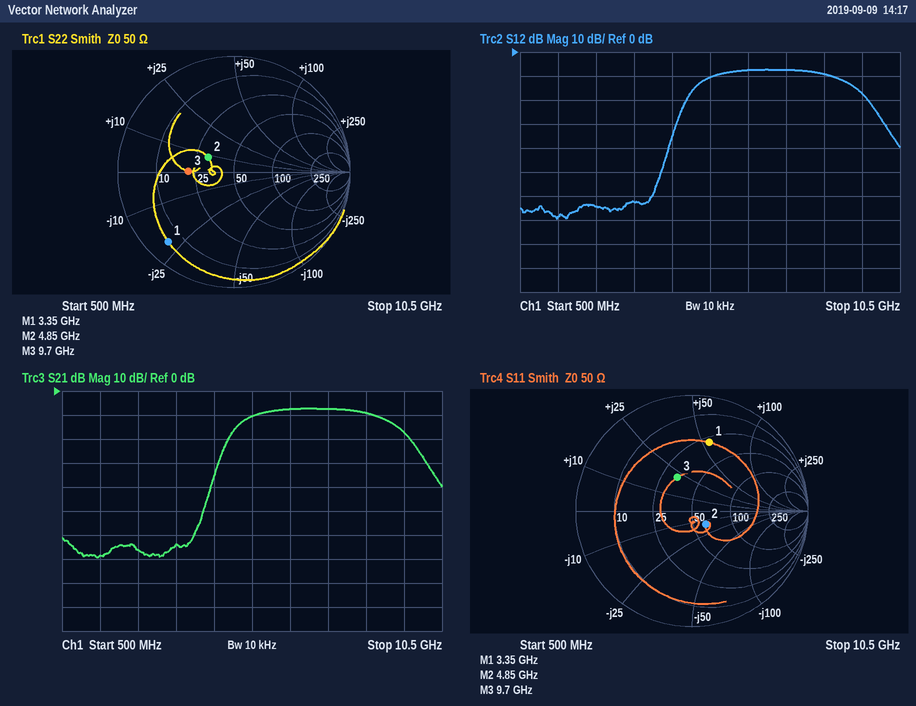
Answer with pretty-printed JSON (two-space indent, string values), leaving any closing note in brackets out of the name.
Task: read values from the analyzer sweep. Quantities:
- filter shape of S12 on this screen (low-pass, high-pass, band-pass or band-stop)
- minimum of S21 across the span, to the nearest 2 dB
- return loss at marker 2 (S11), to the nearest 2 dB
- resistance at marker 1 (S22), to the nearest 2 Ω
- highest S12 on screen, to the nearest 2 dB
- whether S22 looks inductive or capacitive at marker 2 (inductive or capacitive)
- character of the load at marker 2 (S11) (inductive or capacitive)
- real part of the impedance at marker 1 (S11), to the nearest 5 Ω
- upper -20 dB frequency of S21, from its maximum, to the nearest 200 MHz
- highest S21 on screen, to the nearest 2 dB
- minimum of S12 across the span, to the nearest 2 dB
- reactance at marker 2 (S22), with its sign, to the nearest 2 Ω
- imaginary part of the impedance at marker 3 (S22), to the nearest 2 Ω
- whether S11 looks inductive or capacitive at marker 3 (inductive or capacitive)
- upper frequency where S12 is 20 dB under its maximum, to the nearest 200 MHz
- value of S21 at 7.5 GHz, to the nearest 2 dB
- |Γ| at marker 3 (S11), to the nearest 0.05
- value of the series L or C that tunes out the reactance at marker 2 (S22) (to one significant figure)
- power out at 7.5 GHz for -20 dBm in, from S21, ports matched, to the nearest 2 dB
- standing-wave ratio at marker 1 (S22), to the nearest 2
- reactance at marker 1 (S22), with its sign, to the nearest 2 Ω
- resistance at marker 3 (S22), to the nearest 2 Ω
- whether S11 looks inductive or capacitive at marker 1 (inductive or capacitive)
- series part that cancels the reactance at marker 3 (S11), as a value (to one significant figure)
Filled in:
{
  "filter shape of S12 on this screen": "band-pass",
  "minimum of S21 across the span, to the nearest 2 dB": "-70 dB",
  "return loss at marker 2 (S11), to the nearest 2 dB": "16 dB",
  "resistance at marker 1 (S22), to the nearest 2 Ω": "6 Ω",
  "highest S12 on screen, to the nearest 2 dB": "-8 dB",
  "whether S22 looks inductive or capacitive at marker 2": "inductive",
  "character of the load at marker 2 (S11)": "capacitive",
  "real part of the impedance at marker 1 (S11), to the nearest 5 Ω": "30 Ω",
  "upper -20 dB frequency of S21, from its maximum, to the nearest 200 MHz": "10.0 GHz",
  "highest S21 on screen, to the nearest 2 dB": "-8 dB",
  "minimum of S12 across the span, to the nearest 2 dB": "-70 dB",
  "reactance at marker 2 (S22), with its sign, to the nearest 2 Ω": "+8 Ω",
  "imaginary part of the impedance at marker 3 (S22), to the nearest 2 Ω": "0 Ω",
  "whether S11 looks inductive or capacitive at marker 3": "inductive",
  "upper frequency where S12 is 20 dB under its maximum, to the nearest 200 MHz": "10.0 GHz",
  "value of S21 at 7.5 GHz, to the nearest 2 dB": "-8 dB",
  "|Γ| at marker 3 (S11), to the nearest 0.05": "0.30",
  "value of the series L or C that tunes out the reactance at marker 2 (S22)": "4 pF",
  "power out at 7.5 GHz for -20 dBm in, from S21, ports matched, to the nearest 2 dB": "-28 dBm",
  "standing-wave ratio at marker 1 (S22), to the nearest 2": "10",
  "reactance at marker 1 (S22), with its sign, to the nearest 2 Ω": "-22 Ω",
  "resistance at marker 3 (S22), to the nearest 2 Ω": "22 Ω",
  "whether S11 looks inductive or capacitive at marker 1": "inductive",
  "series part that cancels the reactance at marker 3 (S11), as a value": "800 fF"
}
